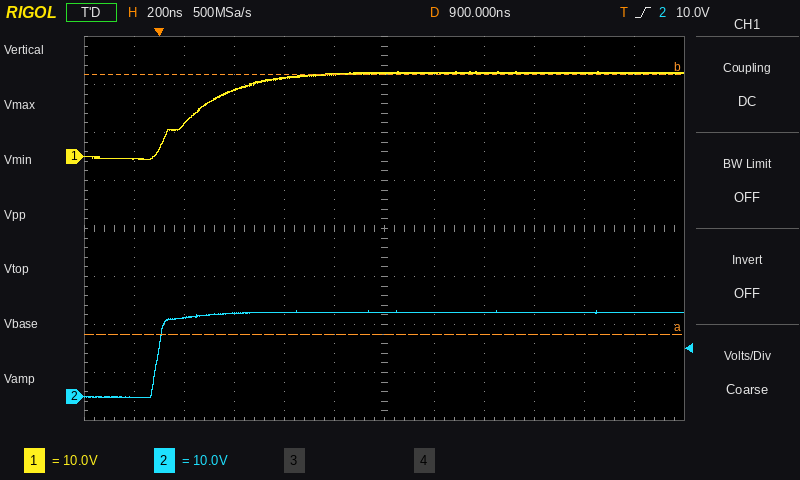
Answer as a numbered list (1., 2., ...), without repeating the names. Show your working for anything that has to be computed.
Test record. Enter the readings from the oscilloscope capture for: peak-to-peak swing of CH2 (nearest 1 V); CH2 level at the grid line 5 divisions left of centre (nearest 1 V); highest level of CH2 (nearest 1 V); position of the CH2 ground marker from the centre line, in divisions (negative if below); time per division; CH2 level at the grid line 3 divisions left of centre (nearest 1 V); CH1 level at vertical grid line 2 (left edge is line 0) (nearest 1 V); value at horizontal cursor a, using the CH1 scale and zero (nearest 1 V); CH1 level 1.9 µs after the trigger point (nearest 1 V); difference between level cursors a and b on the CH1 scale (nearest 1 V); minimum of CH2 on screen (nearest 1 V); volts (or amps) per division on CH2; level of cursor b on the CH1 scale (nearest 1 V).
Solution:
1. 18 V − (0 V) = 18 V
2. 0 V
3. 18 V
4. -3.5 div
5. 200 ns
6. 17 V
7. 7 V
8. -37 V
9. 17 V
10. 54 V
11. 0 V
12. 10 V
13. 17 V
